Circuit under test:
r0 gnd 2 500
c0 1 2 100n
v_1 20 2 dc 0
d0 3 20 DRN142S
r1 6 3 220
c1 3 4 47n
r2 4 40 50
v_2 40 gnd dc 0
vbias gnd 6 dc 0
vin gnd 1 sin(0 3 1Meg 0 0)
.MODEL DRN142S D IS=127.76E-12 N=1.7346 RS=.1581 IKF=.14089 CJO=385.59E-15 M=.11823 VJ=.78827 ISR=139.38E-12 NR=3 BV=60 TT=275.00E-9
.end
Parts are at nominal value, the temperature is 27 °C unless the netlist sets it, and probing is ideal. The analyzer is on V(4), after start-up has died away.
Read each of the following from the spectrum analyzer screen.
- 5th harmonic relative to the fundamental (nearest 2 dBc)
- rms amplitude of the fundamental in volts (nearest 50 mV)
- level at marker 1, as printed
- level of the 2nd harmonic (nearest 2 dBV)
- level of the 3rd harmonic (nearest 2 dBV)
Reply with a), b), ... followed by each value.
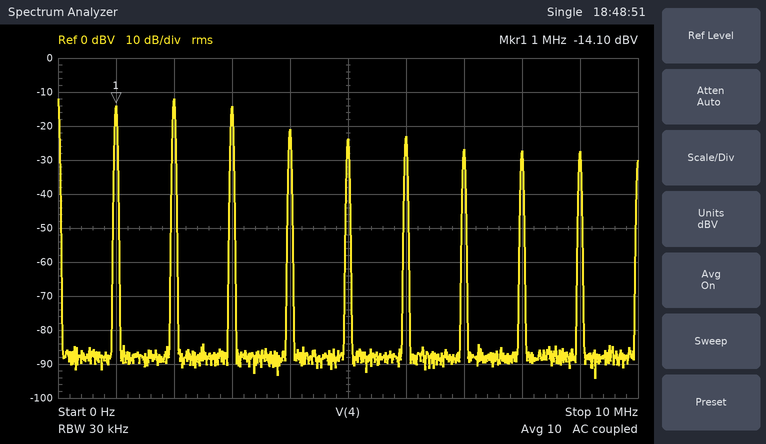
a) -10 dBc
b) 200 mV
c) -14.10 dBV
d) -12 dBV
e) -14 dBV
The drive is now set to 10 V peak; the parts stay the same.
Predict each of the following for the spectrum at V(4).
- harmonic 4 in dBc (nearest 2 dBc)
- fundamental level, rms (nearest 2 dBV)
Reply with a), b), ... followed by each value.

a) -10 dBc
b) -2 dBV
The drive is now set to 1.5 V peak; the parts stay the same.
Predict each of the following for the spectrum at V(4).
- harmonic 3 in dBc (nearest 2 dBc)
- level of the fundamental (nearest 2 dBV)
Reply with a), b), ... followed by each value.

a) 2 dBc
b) -24 dBV
